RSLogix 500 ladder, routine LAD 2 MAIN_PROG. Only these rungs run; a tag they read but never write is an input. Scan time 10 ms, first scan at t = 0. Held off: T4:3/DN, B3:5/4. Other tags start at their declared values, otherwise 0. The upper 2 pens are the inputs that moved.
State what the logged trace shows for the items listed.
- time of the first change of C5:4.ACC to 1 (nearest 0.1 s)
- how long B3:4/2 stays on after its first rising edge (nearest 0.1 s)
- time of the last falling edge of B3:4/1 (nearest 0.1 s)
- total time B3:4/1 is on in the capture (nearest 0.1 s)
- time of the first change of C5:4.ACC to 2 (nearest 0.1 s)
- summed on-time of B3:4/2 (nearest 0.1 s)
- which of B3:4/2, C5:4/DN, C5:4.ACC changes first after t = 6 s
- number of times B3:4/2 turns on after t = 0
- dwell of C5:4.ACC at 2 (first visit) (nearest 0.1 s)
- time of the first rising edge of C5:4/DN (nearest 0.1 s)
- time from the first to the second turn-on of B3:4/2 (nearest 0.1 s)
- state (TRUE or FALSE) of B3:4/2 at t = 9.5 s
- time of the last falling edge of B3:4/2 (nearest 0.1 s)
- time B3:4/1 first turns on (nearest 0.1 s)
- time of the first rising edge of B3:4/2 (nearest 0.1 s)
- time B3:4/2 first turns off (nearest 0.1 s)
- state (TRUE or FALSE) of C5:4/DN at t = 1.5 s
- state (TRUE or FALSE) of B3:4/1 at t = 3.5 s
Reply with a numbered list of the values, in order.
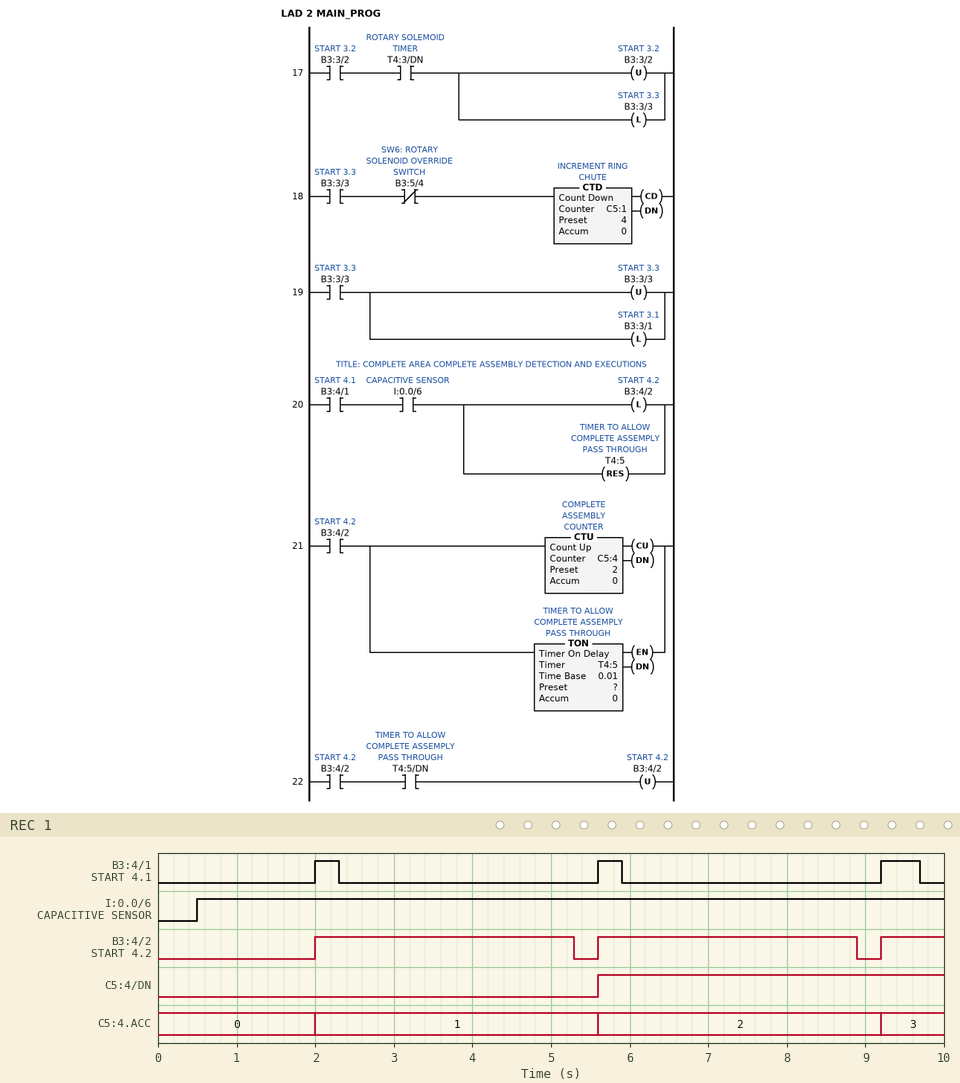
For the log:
1. 2.0 s
2. 3.3 s
3. 9.7 s
4. 1.1 s
5. 5.6 s
6. 7.4 s
7. B3:4/2
8. 3
9. 3.6 s
10. 5.6 s
11. 3.6 s
12. TRUE
13. 8.9 s
14. 2.0 s
15. 2.0 s
16. 5.3 s
17. FALSE
18. FALSE
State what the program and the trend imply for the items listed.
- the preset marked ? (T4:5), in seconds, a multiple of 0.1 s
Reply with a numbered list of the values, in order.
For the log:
1. 3.0 s
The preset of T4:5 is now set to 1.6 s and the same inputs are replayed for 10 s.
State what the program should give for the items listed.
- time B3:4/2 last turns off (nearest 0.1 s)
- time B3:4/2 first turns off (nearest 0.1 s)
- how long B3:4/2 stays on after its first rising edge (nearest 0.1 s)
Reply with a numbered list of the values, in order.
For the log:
1. 7.5 s
2. 3.9 s
3. 1.9 s
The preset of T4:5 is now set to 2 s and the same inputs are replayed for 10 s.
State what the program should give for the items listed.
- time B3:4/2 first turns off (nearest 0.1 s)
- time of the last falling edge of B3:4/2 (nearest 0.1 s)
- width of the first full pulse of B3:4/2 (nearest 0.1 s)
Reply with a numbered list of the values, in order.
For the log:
1. 4.3 s
2. 7.9 s
3. 2.3 s
